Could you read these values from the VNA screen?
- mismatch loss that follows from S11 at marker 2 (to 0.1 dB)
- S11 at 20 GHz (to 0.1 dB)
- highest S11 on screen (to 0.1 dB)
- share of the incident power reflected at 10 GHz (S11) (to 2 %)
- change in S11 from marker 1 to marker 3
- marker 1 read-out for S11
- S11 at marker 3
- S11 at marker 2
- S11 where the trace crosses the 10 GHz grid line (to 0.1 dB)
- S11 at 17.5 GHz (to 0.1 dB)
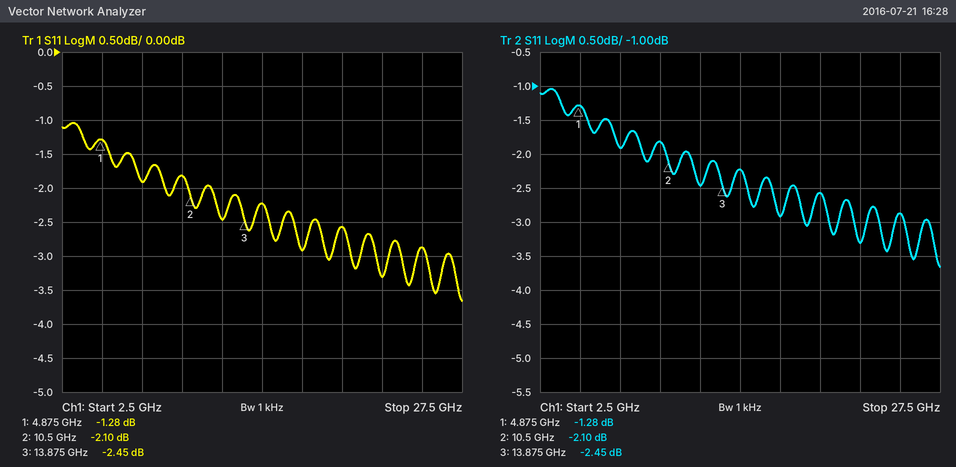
4.2 dB
-2.6 dB
-1.0 dB
66 %
-1.17 dB
-1.28 dB
-2.45 dB
-2.10 dB
-1.8 dB
-2.9 dB
